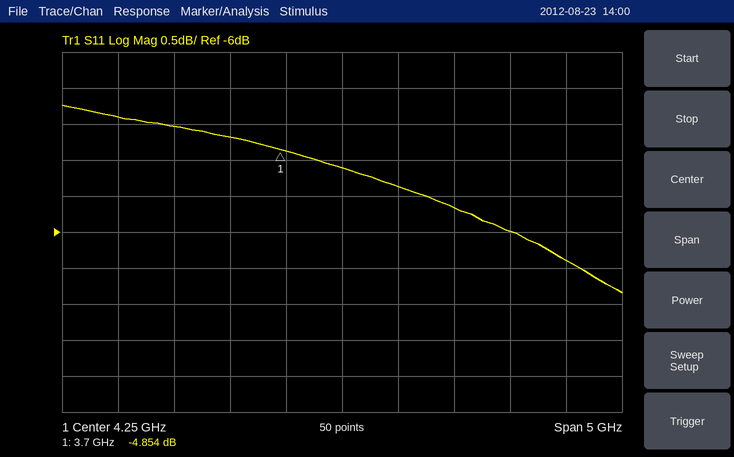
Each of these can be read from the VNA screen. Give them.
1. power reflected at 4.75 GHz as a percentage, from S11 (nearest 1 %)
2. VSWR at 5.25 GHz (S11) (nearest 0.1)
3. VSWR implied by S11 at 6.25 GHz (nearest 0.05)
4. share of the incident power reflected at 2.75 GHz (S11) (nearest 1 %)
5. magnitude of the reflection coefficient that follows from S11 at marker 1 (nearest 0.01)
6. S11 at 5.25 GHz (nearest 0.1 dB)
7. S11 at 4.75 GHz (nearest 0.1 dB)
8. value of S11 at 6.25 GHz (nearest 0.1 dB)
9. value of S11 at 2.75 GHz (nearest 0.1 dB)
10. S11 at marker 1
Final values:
29 %
3.2
2.85
35 %
0.57
-5.7 dB
-5.4 dB
-6.4 dB
-4.5 dB
-4.854 dB
